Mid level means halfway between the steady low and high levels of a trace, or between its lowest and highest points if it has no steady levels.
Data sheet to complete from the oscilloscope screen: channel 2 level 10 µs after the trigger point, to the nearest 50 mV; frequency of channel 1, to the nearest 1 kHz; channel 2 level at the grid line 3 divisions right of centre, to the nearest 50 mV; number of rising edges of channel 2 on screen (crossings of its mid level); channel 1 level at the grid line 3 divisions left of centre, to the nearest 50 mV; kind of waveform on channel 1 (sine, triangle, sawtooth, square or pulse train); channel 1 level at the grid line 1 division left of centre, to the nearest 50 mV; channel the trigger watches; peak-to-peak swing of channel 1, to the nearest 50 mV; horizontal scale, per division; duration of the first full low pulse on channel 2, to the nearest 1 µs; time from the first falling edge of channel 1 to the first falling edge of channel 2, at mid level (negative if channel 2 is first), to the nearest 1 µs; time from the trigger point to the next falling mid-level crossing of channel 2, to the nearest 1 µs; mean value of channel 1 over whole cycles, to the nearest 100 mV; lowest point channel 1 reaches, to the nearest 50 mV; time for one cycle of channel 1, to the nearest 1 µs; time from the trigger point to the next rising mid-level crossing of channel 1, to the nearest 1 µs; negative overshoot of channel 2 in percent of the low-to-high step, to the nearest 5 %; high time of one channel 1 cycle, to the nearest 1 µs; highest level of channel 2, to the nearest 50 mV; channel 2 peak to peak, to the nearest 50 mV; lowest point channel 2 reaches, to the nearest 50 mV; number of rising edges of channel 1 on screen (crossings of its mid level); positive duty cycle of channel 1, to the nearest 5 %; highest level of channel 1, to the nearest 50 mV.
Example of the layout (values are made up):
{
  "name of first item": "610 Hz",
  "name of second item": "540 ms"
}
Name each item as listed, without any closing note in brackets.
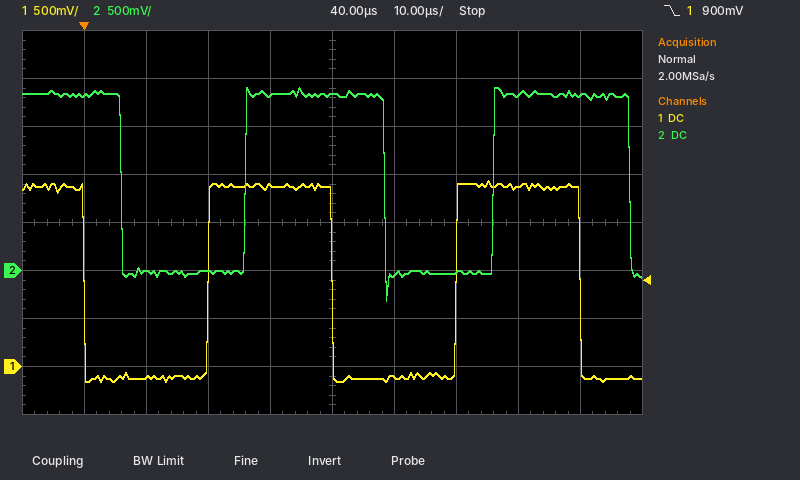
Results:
{
  "channel 2 level 10 µs after the trigger point, to the nearest 50 mV": "0 mV",
  "frequency of channel 1, to the nearest 1 kHz": "25 kHz",
  "channel 2 level at the grid line 3 divisions right of centre, to the nearest 50 mV": "1.85 V",
  "number of rising edges of channel 2 on screen": "2",
  "channel 1 level at the grid line 3 divisions left of centre, to the nearest 50 mV": "-100 mV",
  "kind of waveform on channel 1": "square",
  "channel 1 level at the grid line 1 division left of centre, to the nearest 50 mV": "1.90 V",
  "channel the trigger watches": "channel 1",
  "peak-to-peak swing of channel 1, to the nearest 50 mV": "2.10 V",
  "horizontal scale, per division": "10 µs",
  "duration of the first full low pulse on channel 2, to the nearest 1 µs": "20 µs",
  "time from the first falling edge of channel 1 to the first falling edge of channel 2, at mid level (negative if channel 2 is first), to the nearest 1 µs": "+6 µs",
  "time from the trigger point to the next falling mid-level crossing of channel 2, to the nearest 1 µs": "6 µs",
  "mean value of channel 1 over whole cycles, to the nearest 100 mV": "900 mV",
  "lowest point channel 1 reaches, to the nearest 50 mV": "-150 mV",
  "time for one cycle of channel 1, to the nearest 1 µs": "40 µs",
  "time from the trigger point to the next rising mid-level crossing of channel 1, to the nearest 1 µs": "20 µs",
  "negative overshoot of channel 2 in percent of the low-to-high step, to the nearest 5 %": "15 %",
  "high time of one channel 1 cycle, to the nearest 1 µs": "20 µs",
  "highest level of channel 2, to the nearest 50 mV": "1.90 V",
  "channel 2 peak to peak, to the nearest 50 mV": "2.20 V",
  "lowest point channel 2 reaches, to the nearest 50 mV": "-300 mV",
  "number of rising edges of channel 1 on screen": "2",
  "positive duty cycle of channel 1, to the nearest 5 %": "50 %",
  "highest level of channel 1, to the nearest 50 mV": "1.95 V"
}
